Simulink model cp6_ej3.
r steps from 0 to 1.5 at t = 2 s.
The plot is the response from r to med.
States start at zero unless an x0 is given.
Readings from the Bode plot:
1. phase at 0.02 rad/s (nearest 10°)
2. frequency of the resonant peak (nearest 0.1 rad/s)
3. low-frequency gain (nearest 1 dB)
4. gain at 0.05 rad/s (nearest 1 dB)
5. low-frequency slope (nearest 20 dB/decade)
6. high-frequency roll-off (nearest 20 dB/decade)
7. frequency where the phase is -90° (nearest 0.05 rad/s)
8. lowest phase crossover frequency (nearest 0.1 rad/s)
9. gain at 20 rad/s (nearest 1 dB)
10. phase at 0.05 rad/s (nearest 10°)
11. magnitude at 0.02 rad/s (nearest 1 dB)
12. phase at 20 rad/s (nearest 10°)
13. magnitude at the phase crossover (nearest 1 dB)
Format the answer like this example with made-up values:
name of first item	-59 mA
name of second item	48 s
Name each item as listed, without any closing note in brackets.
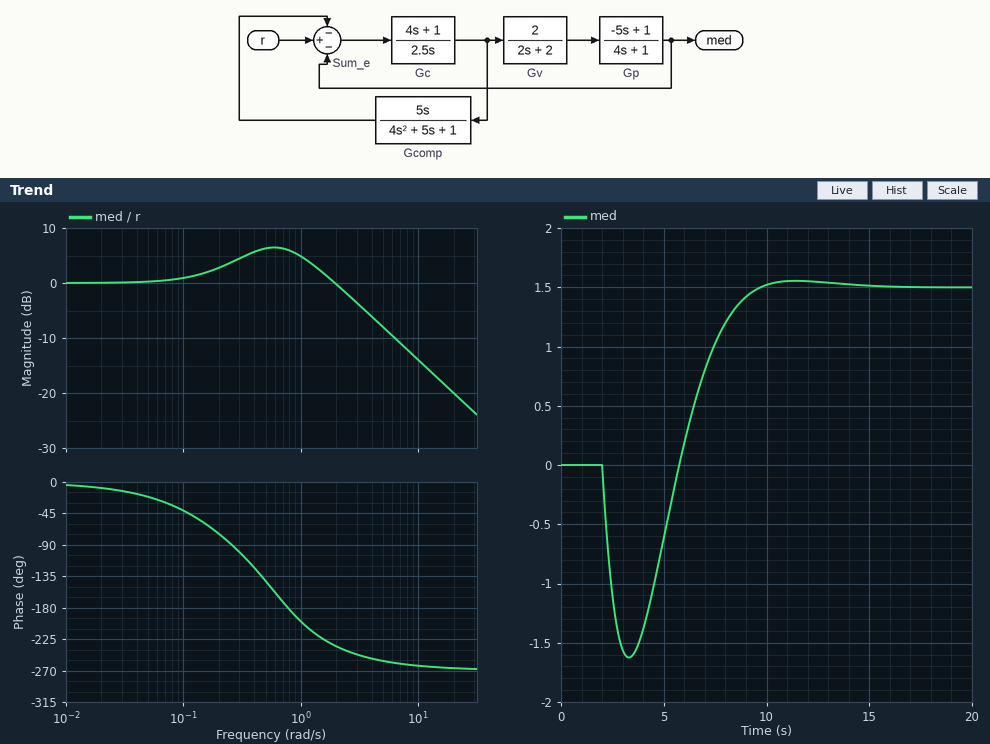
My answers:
phase at 0.02 rad/s	-10°
frequency of the resonant peak	0.6 rad/s
low-frequency gain	0 dB
gain at 0.05 rad/s	0 dB
low-frequency slope	0 dB/decade
high-frequency roll-off	-20 dB/decade
frequency where the phase is -90°	0.25 rad/s
lowest phase crossover frequency	0.8 rad/s
gain at 20 rad/s	-20 dB
phase at 0.05 rad/s	-20°
magnitude at 0.02 rad/s	0 dB
phase at 20 rad/s	-270°
magnitude at the phase crossover	6 dB
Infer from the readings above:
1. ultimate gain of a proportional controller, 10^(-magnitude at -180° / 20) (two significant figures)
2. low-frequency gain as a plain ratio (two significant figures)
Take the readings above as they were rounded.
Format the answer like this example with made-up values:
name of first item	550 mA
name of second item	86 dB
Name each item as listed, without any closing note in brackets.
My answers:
ultimate gain of a proportional controller, 10^(-magnitude at -180° / 20)	0.50
low-frequency gain as a plain ratio	1.0
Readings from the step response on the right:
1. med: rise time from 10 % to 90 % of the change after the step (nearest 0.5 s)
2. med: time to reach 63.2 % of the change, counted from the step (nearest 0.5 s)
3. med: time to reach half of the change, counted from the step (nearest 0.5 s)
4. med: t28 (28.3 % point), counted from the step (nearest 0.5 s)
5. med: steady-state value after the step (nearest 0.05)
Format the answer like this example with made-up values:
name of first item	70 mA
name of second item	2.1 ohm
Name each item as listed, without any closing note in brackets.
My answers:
med: rise time from 10 % to 90 % of the change after the step	2.5 s
med: time to reach 63.2 % of the change, counted from the step	5.5 s
med: time to reach half of the change, counted from the step	5.0 s
med: t28 (28.3 % point), counted from the step	4.5 s
med: steady-state value after the step	1.50
